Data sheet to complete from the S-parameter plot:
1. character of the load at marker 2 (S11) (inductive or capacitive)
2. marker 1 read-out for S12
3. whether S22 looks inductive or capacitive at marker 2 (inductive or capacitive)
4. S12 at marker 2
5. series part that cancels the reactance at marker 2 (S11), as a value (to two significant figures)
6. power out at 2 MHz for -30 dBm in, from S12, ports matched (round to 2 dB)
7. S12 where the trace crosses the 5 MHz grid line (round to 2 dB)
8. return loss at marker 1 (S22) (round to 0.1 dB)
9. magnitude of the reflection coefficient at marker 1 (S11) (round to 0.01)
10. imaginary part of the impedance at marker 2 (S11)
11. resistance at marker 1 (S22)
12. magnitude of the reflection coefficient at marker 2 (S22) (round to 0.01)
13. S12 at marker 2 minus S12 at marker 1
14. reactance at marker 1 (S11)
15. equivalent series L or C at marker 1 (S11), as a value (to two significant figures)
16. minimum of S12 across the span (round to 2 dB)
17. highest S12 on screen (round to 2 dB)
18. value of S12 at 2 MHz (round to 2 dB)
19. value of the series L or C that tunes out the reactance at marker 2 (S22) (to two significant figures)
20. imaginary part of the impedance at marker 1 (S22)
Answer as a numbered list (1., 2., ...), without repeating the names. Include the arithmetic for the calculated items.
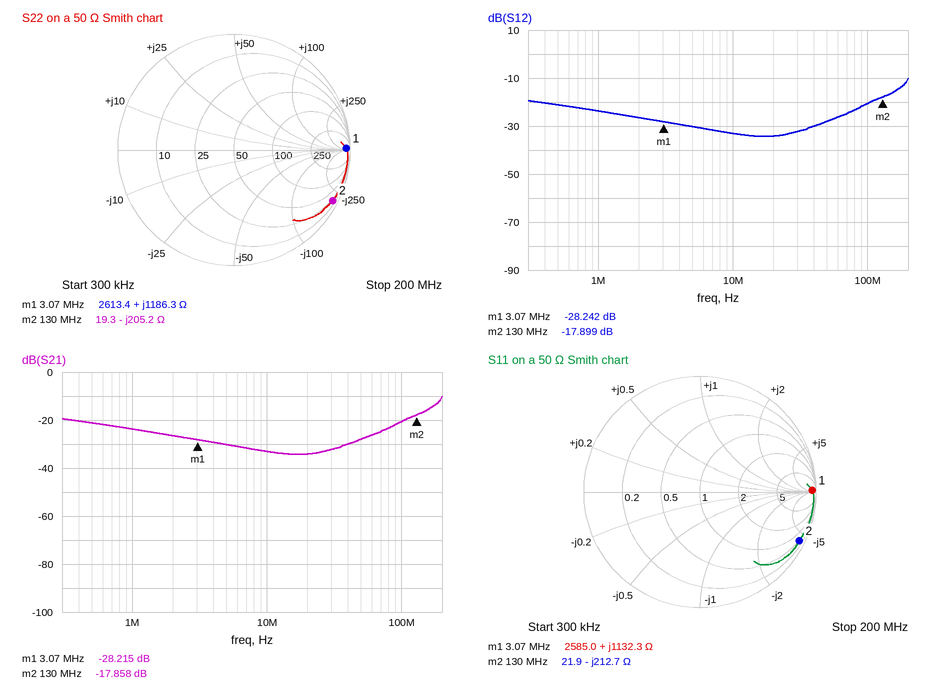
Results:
1. capacitive
2. -28.242 dB
3. capacitive
4. -17.899 dB
5. L = 212.7 Ω/(2π × 130 MHz) ≈ 260 nH
6. -30 dBm + (-26 dB) = -56 dBm
7. -30 dB
8. 0.3 dB
9. 0.97
10. -212.7 Ω
11. 2613.4 Ω
12. 0.96
13. -17.899 − (-28.242) = 10.343 dB
14. +1132.3 Ω
15. L = 1132.3 Ω/(2π × 3.07 MHz) ≈ 59 µH
16. -34 dB
17. -10 dB
18. -26 dB
19. L = 205.2 Ω/(2π × 130 MHz) ≈ 251 nH, so 250 nH to two significant figures
20. +1186.3 Ω
